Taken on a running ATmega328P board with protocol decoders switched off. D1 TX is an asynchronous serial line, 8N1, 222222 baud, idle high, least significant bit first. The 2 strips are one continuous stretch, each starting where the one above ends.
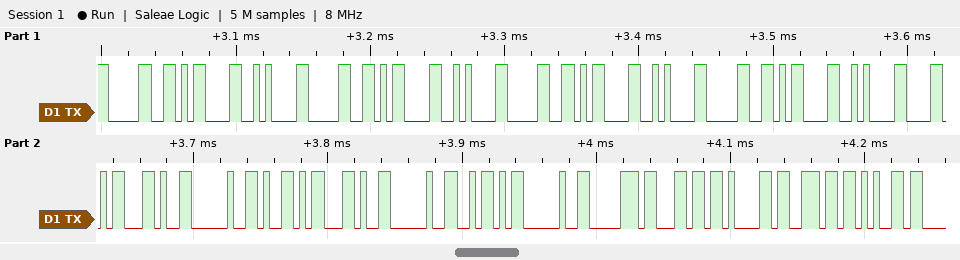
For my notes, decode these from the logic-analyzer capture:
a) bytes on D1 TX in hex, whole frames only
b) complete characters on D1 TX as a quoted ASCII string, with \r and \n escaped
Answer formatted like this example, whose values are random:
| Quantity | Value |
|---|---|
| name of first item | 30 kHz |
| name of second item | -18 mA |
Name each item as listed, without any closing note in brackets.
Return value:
| Quantity | Value |
|---|---|
| bytes on D1 TX in hex, whole frames only | 30 0D 0A 30 0D 0A 30 0D 0A 30 0D 0A 58 2C 20 59 2C 20 5A 20 70 6C 61 6E 65 |
| complete characters on D1 TX as a quoted ASCII string, with \r and \n escaped | "0\r\n0\r\n0\r\n0\r\nX, Y, Z plane" |
